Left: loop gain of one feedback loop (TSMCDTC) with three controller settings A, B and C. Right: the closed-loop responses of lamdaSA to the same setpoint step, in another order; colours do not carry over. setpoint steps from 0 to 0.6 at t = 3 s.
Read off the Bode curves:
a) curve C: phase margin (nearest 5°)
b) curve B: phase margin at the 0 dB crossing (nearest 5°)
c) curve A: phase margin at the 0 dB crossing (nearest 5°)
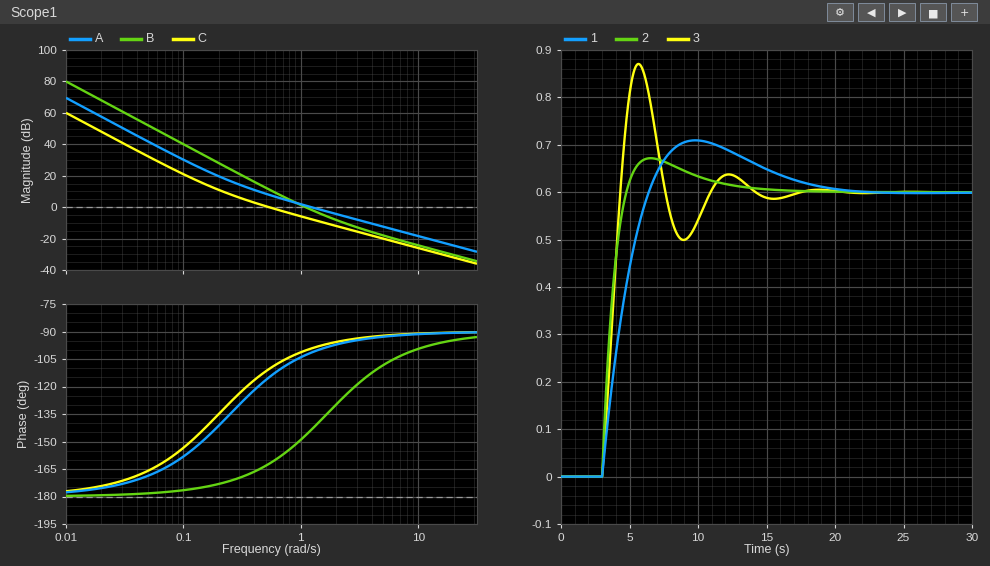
70°
35°
80°
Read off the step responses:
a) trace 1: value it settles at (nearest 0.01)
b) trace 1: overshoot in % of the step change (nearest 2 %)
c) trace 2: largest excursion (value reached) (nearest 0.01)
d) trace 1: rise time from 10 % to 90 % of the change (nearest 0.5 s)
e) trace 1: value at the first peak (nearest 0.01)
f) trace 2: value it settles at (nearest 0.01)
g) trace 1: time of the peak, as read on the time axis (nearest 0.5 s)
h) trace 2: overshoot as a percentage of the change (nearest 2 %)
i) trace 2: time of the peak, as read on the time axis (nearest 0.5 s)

0.60
18 %
0.67
2.5 s
0.71
0.60
10.0 s
12 %
6.5 s
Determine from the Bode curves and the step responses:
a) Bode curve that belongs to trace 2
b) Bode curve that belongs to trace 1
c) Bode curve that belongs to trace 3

A
C
B
